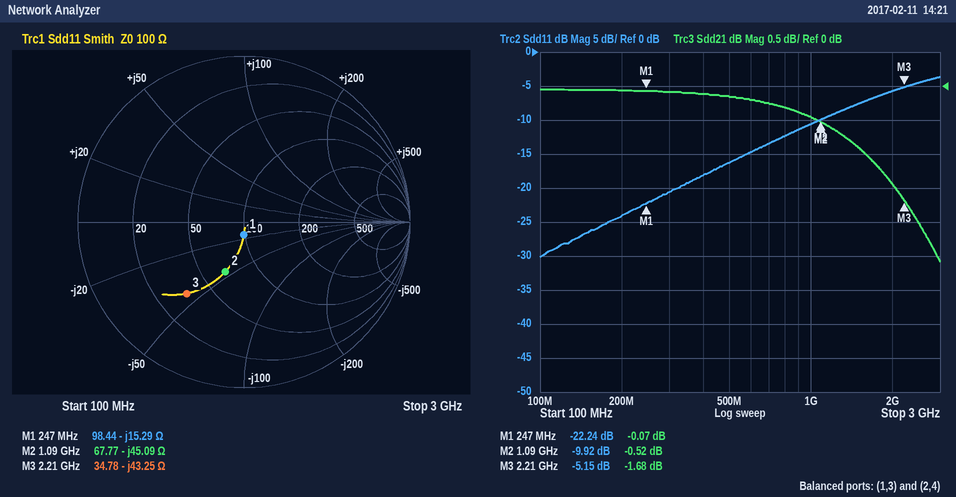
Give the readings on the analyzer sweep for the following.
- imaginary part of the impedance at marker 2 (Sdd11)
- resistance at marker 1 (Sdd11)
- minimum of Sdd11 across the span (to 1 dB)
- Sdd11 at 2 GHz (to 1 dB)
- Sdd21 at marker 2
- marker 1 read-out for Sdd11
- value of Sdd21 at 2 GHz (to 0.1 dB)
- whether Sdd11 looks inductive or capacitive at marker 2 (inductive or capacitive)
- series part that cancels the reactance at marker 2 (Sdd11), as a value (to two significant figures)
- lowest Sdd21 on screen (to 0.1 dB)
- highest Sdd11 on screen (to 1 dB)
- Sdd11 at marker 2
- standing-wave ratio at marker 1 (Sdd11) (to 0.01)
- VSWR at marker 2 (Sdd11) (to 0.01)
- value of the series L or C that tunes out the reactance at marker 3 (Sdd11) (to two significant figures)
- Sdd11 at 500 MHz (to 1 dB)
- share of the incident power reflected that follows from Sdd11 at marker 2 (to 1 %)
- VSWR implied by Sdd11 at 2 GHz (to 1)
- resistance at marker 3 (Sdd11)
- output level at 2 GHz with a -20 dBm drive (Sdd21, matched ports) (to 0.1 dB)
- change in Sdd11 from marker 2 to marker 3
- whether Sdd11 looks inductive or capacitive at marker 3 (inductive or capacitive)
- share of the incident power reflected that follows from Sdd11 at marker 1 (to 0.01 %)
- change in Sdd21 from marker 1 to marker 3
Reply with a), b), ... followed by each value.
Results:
a) -45.09 Ω
b) 98.44 Ω
c) -30 dB
d) -6 dB
e) -0.52 dB
f) -22.24 dB
g) -1.4 dB
h) capacitive
i) 6.6 nH
j) -2.6 dB
k) -4 dB
l) -9.92 dB
m) 1.17
n) 1.94
o) 3.1 nH
p) -16 dB
q) 10 %
r) 3
s) 34.78 Ω
t) -21.4 dBm
u) 4.77 dB
v) capacitive
w) 0.60 %
x) -1.61 dB
